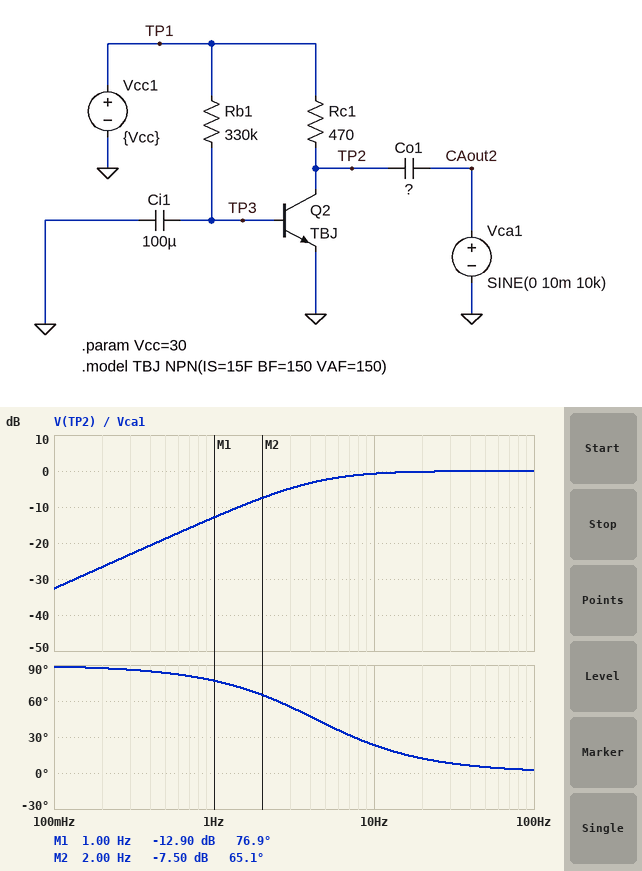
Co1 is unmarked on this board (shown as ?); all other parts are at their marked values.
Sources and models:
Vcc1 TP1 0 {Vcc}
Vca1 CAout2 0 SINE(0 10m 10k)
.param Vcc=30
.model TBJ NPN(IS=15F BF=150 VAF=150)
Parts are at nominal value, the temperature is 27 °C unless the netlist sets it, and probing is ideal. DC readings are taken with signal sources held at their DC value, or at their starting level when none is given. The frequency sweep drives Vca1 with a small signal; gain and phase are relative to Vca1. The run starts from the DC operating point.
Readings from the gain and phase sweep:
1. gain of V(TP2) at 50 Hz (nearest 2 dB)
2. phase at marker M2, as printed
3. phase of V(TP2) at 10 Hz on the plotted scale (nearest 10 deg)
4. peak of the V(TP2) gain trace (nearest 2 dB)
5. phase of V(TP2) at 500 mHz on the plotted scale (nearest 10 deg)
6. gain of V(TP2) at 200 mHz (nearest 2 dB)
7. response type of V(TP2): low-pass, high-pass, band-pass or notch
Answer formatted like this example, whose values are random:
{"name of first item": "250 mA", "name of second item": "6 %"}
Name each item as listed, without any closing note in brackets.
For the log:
{"gain of V(TP2) at 50 Hz": "0 dB", "phase at marker M2, as printed": "65.1 deg", "phase of V(TP2) at 10 Hz on the plotted scale": "20 deg", "peak of the V(TP2) gain trace": "0 dB", "phase of V(TP2) at 500 mHz on the plotted scale": "80 deg", "gain of V(TP2) at 200 mHz": "-26 dB", "response type of V(TP2): low-pass, high-pass, band-pass or notch": "high-pass"}
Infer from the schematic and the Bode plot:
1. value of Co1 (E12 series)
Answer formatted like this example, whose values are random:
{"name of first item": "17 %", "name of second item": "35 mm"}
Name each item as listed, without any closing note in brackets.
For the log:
{"value of Co1": "82 µF"}
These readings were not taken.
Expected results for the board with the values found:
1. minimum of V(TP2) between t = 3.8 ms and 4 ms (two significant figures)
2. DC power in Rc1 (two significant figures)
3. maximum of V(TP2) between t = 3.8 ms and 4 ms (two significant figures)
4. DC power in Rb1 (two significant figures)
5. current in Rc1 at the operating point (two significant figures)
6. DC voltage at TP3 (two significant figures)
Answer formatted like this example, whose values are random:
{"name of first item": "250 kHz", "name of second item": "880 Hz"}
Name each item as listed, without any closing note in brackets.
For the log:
{"minimum of V(TP2) between t = 3.8 ms and 4 ms": "23 V", "DC power in Rc1": "110 mW", "maximum of V(TP2) between t = 3.8 ms and 4 ms": "23 V", "DC power in Rb1": "2.6 mW", "current in Rc1 at the operating point": "15 mA", "DC voltage at TP3": "710 mV"}
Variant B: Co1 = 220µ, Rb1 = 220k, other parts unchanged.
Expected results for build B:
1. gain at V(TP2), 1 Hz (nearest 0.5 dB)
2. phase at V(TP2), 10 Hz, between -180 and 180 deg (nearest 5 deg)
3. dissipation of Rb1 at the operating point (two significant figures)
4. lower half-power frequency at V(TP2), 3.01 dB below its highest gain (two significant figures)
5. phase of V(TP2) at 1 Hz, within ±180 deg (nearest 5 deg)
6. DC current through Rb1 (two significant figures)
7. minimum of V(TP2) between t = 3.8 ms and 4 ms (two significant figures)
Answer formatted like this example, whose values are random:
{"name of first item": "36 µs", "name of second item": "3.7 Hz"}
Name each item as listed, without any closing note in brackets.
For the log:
{"gain at V(TP2), 1 Hz": "-5.5 dB", "phase at V(TP2), 10 Hz, between -180 and 180 deg": "10 deg", "dissipation of Rb1 at the operating point": "3.9 mW", "lower half-power frequency at V(TP2), 3.01 dB below its highest gain": "1.6 Hz", "phase of V(TP2) at 1 Hz, within ±180 deg": "60 deg", "DC current through Rb1": "130 µA", "minimum of V(TP2) between t = 3.8 ms and 4 ms": "19 V"}
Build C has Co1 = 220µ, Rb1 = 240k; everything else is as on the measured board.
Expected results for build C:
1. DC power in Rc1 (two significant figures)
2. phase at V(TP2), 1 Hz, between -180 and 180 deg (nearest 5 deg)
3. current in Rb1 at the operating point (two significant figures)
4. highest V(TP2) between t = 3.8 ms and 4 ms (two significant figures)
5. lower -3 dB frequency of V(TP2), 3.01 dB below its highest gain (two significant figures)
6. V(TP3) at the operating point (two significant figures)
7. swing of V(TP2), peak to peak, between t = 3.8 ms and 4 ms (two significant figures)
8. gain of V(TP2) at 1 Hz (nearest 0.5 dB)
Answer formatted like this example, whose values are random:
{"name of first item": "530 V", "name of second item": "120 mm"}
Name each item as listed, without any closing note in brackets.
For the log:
{"DC power in Rc1": "200 mW", "phase at V(TP2), 1 Hz, between -180 and 180 deg": "60 deg", "current in Rb1 at the operating point": "120 µA", "highest V(TP2) between t = 3.8 ms and 4 ms": "20 V", "lower -3 dB frequency of V(TP2), 3.01 dB below its highest gain": "1.6 Hz", "V(TP3) at the operating point": "720 mV", "swing of V(TP2), peak to peak, between t = 3.8 ms and 4 ms": "20 mV", "gain of V(TP2) at 1 Hz": "-5.5 dB"}
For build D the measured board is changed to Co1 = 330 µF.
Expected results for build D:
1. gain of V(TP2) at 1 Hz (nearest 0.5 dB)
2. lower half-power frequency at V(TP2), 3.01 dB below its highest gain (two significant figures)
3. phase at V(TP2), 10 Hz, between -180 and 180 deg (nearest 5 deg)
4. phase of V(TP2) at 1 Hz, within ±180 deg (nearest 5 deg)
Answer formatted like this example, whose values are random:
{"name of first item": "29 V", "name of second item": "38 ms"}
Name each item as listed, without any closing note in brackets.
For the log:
{"gain of V(TP2) at 1 Hz": "-3.5 dB", "lower half-power frequency at V(TP2), 3.01 dB below its highest gain": "1.1 Hz", "phase at V(TP2), 10 Hz, between -180 and 180 deg": "5 deg", "phase of V(TP2) at 1 Hz, within ±180 deg": "45 deg"}
